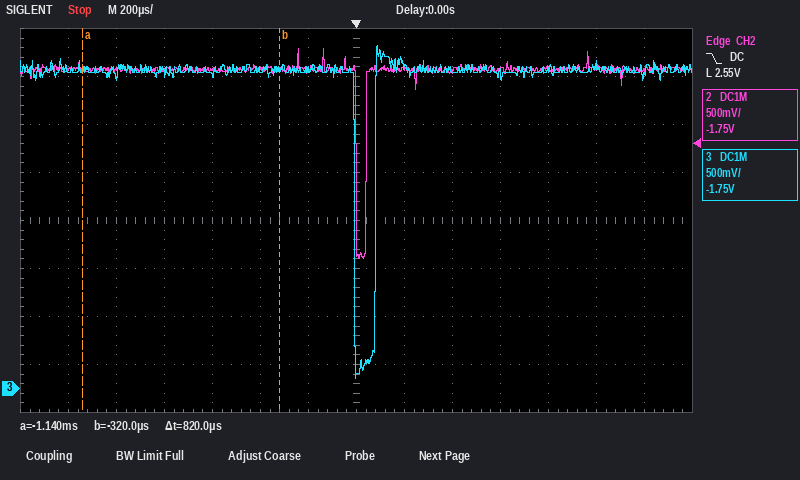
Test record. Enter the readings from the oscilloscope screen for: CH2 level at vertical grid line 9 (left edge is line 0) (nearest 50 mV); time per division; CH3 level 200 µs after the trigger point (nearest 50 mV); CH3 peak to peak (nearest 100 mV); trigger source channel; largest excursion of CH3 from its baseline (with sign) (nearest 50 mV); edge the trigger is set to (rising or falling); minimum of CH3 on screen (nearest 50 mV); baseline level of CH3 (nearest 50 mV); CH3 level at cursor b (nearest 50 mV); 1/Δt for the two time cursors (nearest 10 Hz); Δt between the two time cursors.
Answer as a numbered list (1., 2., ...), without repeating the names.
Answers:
1. 3.30 V
2. 200 µs
3. 3.35 V
4. 3.50 V
5. CH2
6. -3.20 V
7. falling
8. 100 mV
9. 3.30 V
10. 3.35 V
11. 1.22 kHz
12. 820 µs
